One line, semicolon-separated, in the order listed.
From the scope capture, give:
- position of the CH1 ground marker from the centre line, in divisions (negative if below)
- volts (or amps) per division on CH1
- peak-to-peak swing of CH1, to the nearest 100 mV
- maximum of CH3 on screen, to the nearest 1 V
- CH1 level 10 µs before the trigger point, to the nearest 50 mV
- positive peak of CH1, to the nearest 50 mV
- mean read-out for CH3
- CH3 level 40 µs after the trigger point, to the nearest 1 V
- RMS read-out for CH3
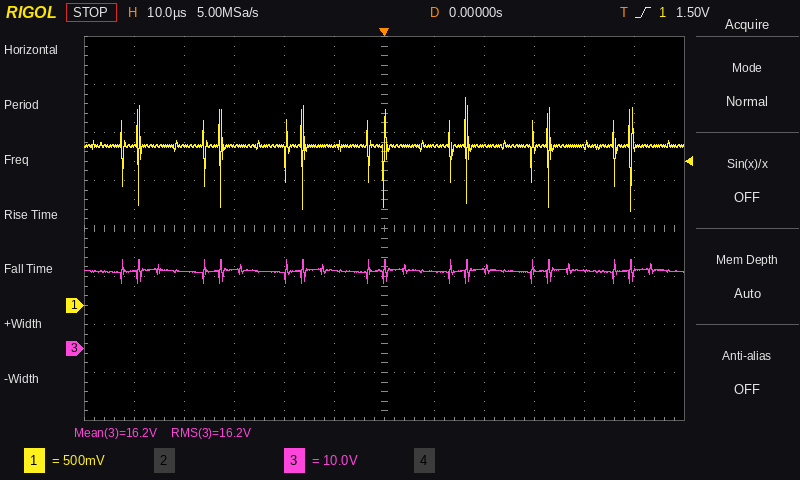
-1.6 div; 500 mV; 1.20 V; 19 V; 1.65 V; 2.15 V; 16.2 V; 16 V; 16.2 V
